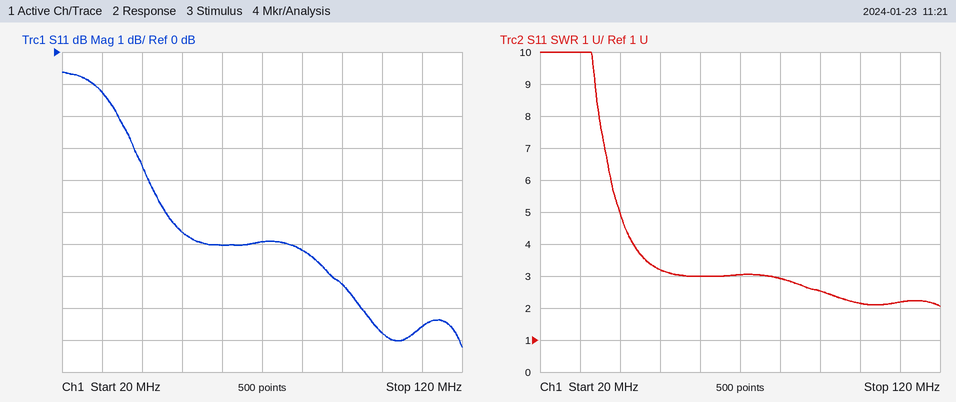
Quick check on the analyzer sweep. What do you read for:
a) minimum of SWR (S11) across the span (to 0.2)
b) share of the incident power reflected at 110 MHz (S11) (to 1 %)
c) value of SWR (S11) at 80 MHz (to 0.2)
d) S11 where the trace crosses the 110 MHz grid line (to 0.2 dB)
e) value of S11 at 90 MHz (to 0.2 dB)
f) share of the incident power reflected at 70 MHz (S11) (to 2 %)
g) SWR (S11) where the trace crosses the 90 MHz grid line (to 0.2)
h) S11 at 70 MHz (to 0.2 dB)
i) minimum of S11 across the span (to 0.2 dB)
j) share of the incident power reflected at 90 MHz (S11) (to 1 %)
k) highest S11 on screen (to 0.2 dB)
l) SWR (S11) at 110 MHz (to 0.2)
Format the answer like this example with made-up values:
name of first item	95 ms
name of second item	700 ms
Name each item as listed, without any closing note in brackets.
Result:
minimum of SWR (S11) across the span	2.0
share of the incident power reflected at 110 MHz (S11)	14 %
value of SWR (S11) at 80 MHz	3.0
S11 where the trace crosses the 110 MHz grid line	-8.6 dB
value of S11 at 90 MHz	-7.2 dB
share of the incident power reflected at 70 MHz (S11)	26 %
SWR (S11) where the trace crosses the 90 MHz grid line	2.6
S11 at 70 MHz	-6.0 dB
minimum of S11 across the span	-9.2 dB
share of the incident power reflected at 90 MHz (S11)	19 %
highest S11 on screen	-0.6 dB
SWR (S11) at 110 MHz	2.2
